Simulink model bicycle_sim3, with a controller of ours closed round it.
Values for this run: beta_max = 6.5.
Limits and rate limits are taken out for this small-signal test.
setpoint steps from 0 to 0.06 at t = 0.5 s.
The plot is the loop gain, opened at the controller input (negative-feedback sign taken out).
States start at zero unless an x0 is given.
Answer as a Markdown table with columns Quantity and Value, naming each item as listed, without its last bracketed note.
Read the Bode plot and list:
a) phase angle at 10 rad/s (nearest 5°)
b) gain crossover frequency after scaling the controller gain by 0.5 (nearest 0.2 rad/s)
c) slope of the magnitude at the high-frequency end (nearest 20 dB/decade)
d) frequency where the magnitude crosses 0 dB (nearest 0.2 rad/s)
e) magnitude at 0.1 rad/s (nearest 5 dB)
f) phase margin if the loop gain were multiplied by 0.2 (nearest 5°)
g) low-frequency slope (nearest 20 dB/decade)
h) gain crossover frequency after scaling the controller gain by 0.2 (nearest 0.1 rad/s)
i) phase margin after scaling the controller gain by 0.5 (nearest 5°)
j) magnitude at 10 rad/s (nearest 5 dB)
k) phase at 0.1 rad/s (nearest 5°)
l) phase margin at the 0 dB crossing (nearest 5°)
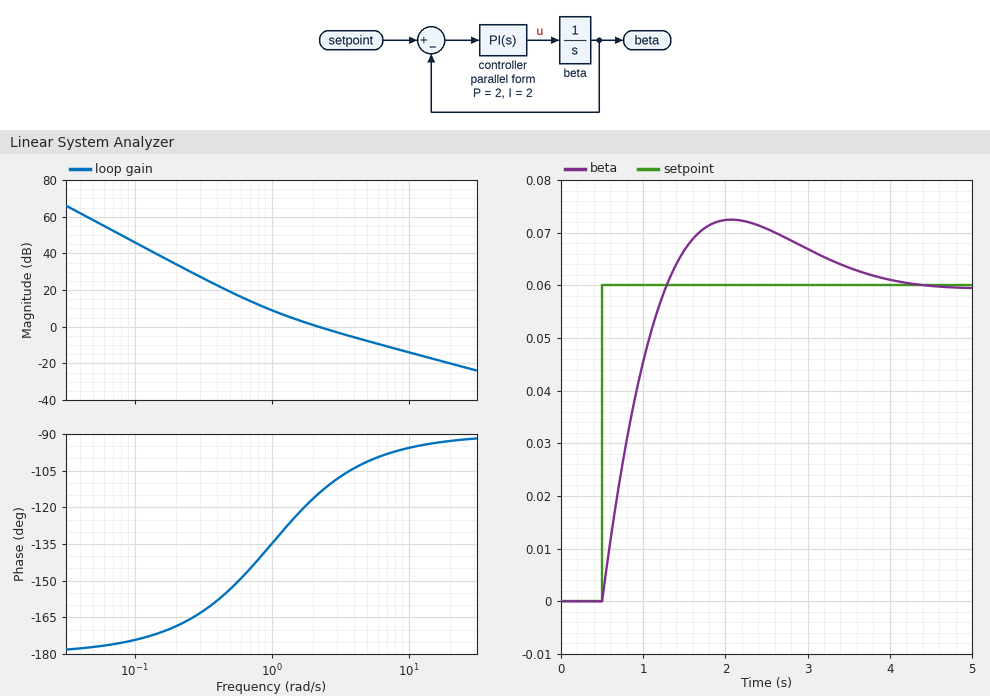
| Quantity | Value |
|---|---|
| phase angle at 10 rad/s | -95° |
| gain crossover frequency after scaling the controller gain by 0.5 | 1.2 rad/s |
| slope of the magnitude at the high-frequency end | -20 dB/decade |
| frequency where the magnitude crosses 0 dB | 2.2 rad/s |
| magnitude at 0.1 rad/s | 45 dB |
| phase margin if the loop gain were multiplied by 0.2 | 35° |
| low-frequency slope | -40 dB/decade |
| gain crossover frequency after scaling the controller gain by 0.2 | 0.7 rad/s |
| phase margin after scaling the controller gain by 0.5 | 50° |
| magnitude at 10 rad/s | -15 dB |
| phase at 0.1 rad/s | -175° |
| phase margin at the 0 dB crossing | 65° |
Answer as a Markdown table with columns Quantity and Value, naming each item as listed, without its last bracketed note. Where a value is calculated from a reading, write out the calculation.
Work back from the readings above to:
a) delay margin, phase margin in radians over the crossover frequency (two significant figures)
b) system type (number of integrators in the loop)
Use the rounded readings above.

| Quantity | Value |
|---|---|
| delay margin, phase margin in radians over the crossover frequency | 65 × π / 180 / 2.2 = 0.52 s |
| system type | 2 |
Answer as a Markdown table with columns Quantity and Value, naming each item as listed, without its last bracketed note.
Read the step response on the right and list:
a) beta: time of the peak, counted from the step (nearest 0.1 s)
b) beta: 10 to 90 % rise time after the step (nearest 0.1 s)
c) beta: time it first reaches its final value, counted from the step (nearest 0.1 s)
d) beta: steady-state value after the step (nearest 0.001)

| Quantity | Value |
|---|---|
| beta: time of the peak, counted from the step | 1.6 s |
| beta: 10 to 90 % rise time after the step | 0.6 s |
| beta: time it first reaches its final value, counted from the step | 0.8 s |
| beta: steady-state value after the step | 0.060 |
